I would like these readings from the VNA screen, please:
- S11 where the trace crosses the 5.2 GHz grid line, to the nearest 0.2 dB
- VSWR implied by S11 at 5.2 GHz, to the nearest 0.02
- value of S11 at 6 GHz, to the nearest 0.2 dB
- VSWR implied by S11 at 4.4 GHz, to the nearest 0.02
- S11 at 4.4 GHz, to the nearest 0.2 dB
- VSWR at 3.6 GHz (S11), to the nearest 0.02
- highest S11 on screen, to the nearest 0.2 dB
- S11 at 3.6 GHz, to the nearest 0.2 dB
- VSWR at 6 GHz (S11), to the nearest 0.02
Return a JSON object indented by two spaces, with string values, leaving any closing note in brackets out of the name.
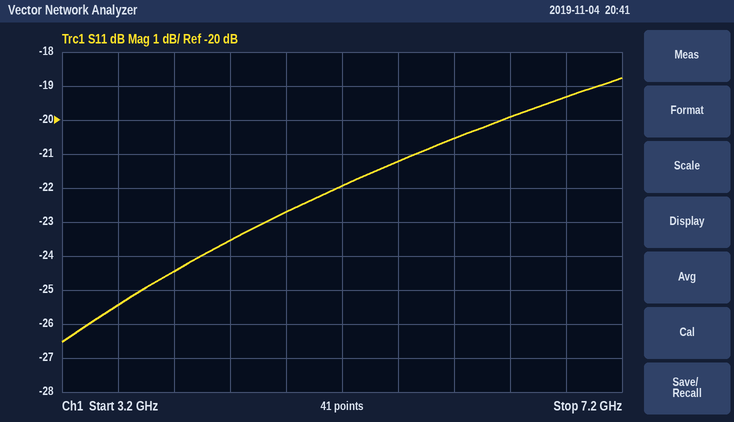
{
  "S11 where the trace crosses the 5.2 GHz grid line, to the nearest 0.2 dB": "-22.0 dB",
  "VSWR implied by S11 at 5.2 GHz, to the nearest 0.02": "1.18",
  "value of S11 at 6 GHz, to the nearest 0.2 dB": "-20.6 dB",
  "VSWR implied by S11 at 4.4 GHz, to the nearest 0.02": "1.14",
  "S11 at 4.4 GHz, to the nearest 0.2 dB": "-23.6 dB",
  "VSWR at 3.6 GHz (S11), to the nearest 0.02": "1.12",
  "highest S11 on screen, to the nearest 0.2 dB": "-18.8 dB",
  "S11 at 3.6 GHz, to the nearest 0.2 dB": "-25.4 dB",
  "VSWR at 6 GHz (S11), to the nearest 0.02": "1.20"
}
